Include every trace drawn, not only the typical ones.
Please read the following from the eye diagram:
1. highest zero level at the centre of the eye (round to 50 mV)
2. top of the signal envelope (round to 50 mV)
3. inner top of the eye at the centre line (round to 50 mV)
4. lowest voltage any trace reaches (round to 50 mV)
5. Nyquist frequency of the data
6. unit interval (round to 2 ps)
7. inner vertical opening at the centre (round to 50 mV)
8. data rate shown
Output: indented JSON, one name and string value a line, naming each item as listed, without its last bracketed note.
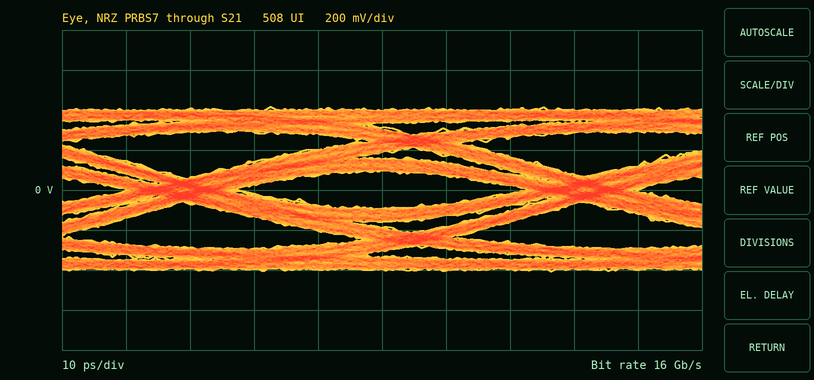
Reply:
{
  "highest zero level at the centre of the eye": "-100 mV",
  "top of the signal envelope": "400 mV",
  "inner top of the eye at the centre line": "100 mV",
  "lowest voltage any trace reaches": "-400 mV",
  "Nyquist frequency of the data": "8 GHz",
  "unit interval": "62 ps",
  "inner vertical opening at the centre": "200 mV",
  "data rate shown": "16 Gb/s"
}
